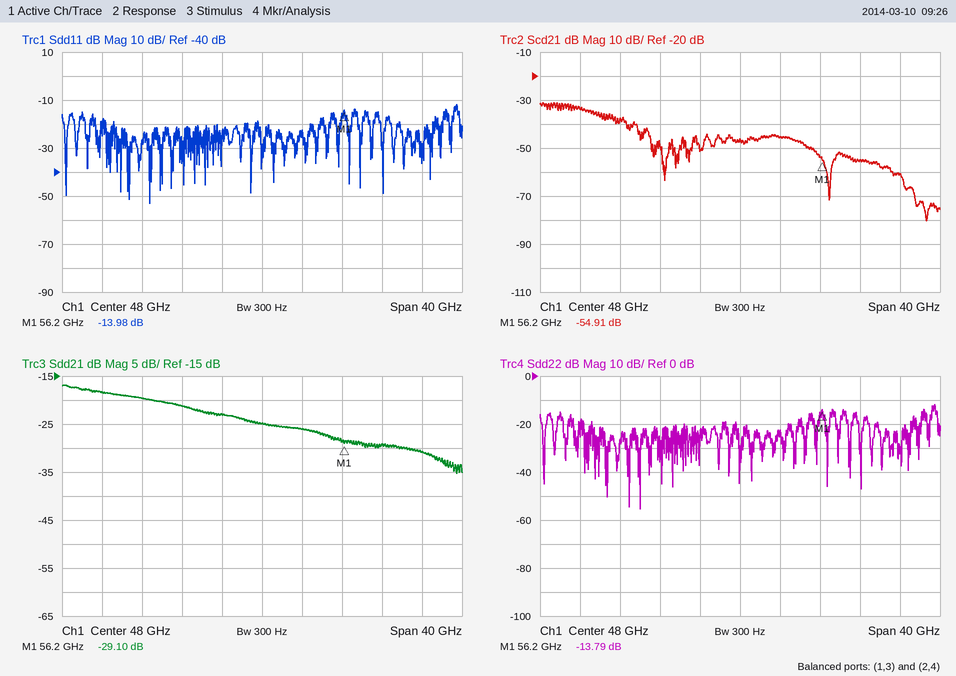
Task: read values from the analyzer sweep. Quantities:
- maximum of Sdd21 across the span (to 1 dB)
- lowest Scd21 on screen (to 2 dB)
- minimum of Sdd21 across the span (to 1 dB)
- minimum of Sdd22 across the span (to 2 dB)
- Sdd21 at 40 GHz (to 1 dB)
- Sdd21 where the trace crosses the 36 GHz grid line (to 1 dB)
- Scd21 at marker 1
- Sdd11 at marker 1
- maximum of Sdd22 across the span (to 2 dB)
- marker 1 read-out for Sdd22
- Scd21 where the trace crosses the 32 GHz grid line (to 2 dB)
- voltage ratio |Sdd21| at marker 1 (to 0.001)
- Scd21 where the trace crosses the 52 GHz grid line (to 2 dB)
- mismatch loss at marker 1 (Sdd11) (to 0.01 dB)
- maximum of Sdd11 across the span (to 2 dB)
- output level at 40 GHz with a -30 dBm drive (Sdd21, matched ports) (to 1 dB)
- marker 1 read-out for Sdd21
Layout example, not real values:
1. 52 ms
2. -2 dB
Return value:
1. -17 dB
2. -80 dB
3. -35 dB
4. -56 dB
5. -21 dB
6. -20 dB
7. -54.91 dB
8. -13.98 dB
9. -12 dB
10. -13.79 dB
11. -34 dB
12. 0.035
13. -46 dB
14. 0.18 dB
15. -12 dB
16. -51 dBm
17. -29.10 dB
